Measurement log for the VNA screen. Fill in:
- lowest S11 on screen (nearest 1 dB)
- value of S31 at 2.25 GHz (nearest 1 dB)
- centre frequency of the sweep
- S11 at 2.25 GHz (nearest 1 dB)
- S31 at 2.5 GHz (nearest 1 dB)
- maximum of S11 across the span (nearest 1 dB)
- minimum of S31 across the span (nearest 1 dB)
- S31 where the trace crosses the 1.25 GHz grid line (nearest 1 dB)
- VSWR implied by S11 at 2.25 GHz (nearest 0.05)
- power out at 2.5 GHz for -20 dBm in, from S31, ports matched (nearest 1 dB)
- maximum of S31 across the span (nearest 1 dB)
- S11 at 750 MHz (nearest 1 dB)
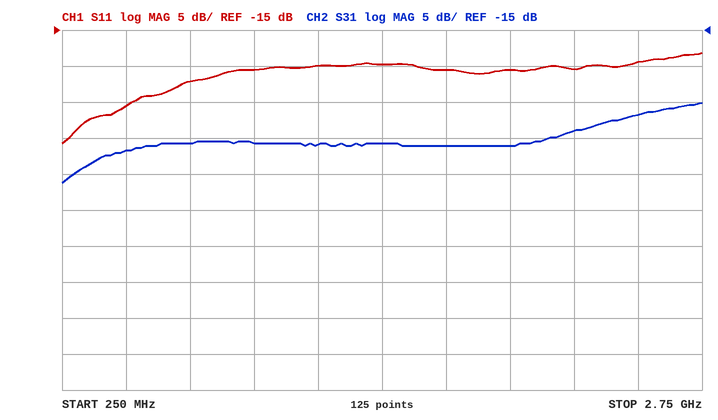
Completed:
-31 dB
-29 dB
1.5 GHz
-20 dB
-27 dB
-18 dB
-36 dB
-31 dB
1.20
-47 dBm
-25 dB
-22 dB
